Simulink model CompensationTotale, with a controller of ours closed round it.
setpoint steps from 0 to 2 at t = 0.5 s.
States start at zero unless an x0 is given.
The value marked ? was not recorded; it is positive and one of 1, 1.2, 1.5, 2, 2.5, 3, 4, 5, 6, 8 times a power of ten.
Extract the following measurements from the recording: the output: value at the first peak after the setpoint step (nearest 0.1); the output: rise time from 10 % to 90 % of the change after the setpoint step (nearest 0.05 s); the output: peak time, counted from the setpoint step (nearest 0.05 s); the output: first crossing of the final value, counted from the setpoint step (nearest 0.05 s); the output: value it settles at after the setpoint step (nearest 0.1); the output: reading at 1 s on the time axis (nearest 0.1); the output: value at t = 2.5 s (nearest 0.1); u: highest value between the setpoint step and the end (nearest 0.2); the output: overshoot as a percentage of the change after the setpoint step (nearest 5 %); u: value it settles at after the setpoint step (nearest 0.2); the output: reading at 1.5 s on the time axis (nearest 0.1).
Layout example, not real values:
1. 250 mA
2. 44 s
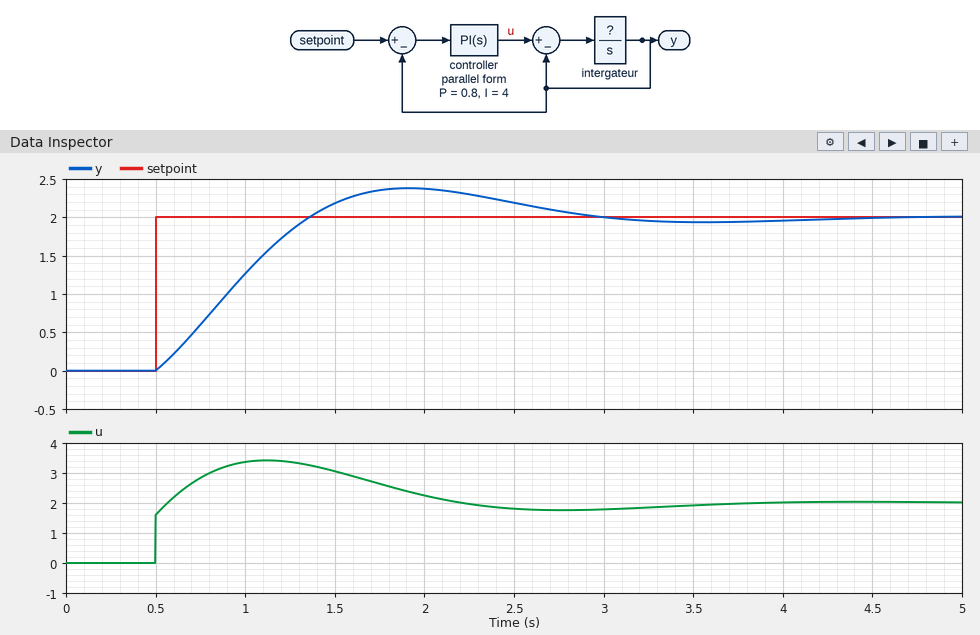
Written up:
1. 2.4
2. 0.65 s
3. 1.40 s
4. 0.85 s
5. 2.0
6. 1.3
7. 2.2
8. 3.4
9. 20 %
10. 2.0
11. 2.2
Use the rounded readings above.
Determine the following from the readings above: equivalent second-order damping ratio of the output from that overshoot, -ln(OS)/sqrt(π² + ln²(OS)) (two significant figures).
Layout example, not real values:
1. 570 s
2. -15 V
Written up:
1. 0.46
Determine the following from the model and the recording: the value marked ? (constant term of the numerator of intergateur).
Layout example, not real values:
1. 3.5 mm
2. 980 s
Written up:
1. 1.2
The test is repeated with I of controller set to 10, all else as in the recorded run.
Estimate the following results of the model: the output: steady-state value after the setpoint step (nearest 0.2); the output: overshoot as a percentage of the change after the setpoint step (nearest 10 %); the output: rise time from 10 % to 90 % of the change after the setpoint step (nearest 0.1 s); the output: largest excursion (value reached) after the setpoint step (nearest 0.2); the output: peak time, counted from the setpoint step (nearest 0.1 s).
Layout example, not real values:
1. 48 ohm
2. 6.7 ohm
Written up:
1. 2.0
2. 40 %
3. 0.4 s
4. 2.8
5. 0.9 s
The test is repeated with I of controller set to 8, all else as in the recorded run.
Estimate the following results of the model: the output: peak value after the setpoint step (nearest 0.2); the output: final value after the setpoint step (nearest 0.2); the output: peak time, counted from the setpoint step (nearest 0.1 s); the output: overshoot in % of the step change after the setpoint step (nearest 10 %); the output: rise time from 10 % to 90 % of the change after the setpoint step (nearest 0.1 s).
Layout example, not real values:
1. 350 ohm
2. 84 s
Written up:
1. 2.6
2. 2.0
3. 1.0 s
4. 30 %
5. 0.4 s
